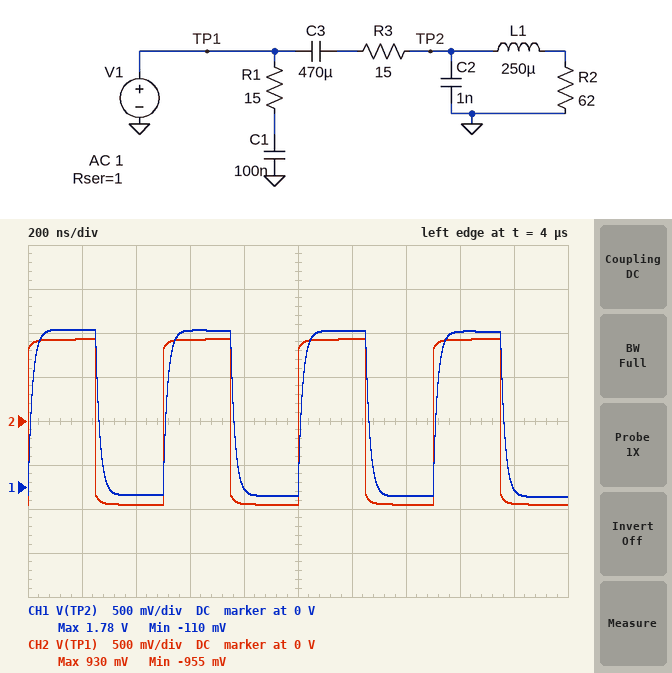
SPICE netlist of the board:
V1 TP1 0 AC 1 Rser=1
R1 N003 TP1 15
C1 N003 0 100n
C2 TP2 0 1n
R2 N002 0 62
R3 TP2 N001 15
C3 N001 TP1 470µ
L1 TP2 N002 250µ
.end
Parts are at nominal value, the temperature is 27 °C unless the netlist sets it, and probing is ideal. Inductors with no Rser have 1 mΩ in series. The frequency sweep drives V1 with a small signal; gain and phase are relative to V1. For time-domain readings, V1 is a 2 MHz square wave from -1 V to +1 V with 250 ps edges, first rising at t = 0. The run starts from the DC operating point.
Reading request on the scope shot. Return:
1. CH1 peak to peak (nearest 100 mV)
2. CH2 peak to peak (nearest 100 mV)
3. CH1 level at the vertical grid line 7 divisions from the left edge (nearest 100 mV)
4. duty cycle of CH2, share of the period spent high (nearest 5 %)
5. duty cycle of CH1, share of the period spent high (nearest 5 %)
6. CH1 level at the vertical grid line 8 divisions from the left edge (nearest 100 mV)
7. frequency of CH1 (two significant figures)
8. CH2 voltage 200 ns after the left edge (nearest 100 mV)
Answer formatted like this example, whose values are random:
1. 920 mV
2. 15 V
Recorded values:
1. 1.9 V
2. 1.9 V
3. -100 mV
4. 50 %
5. 50 %
6. 1.8 V
7. 2.0 MHz
8. 900 mV
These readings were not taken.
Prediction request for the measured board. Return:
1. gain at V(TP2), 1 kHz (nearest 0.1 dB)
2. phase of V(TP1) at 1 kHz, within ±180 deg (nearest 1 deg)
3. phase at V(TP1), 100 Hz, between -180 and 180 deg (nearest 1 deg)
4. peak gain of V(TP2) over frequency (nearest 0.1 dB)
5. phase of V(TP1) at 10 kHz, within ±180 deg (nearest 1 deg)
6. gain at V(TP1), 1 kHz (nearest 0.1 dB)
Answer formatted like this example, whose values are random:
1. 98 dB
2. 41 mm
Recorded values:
1. -2.0 dB
2. 0 deg
3. 0 deg
4. -0.5 dB
5. 0 deg
6. -0.1 dB
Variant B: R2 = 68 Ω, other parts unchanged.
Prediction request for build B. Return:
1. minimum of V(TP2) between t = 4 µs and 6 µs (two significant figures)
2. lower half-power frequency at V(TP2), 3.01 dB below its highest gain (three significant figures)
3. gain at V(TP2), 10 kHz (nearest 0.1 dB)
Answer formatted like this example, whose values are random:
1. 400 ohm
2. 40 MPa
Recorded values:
1. -100 mV
2. 5.80 Hz
3. -1.8 dB
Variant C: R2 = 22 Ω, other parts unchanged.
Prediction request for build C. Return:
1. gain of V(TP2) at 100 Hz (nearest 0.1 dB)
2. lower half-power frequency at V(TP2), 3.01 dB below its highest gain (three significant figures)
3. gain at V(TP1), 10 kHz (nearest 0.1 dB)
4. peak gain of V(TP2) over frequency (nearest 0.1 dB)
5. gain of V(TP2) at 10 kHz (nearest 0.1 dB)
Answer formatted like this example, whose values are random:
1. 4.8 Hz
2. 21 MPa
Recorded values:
1. -4.8 dB
2. 11.3 kHz
3. -0.2 dB
4. -0.4 dB
5. -3.6 dB
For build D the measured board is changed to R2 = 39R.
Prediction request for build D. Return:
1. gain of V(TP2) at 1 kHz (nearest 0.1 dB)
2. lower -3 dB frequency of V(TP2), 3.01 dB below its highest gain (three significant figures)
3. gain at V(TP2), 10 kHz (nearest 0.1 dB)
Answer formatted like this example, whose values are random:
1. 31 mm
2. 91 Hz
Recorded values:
1. -3.0 dB
2. 17.4 Hz
3. -2.7 dB
